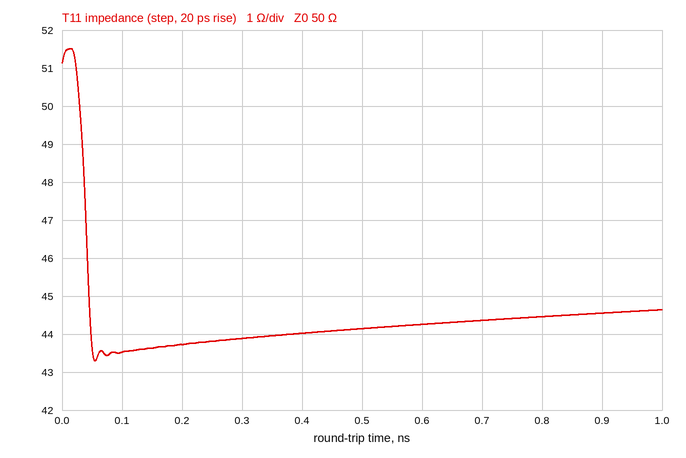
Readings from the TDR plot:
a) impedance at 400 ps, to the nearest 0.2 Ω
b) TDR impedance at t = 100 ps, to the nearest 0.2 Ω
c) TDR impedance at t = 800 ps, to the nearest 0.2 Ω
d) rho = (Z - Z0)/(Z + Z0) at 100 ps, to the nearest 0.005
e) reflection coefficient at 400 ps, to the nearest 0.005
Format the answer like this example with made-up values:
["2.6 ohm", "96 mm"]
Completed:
["44.0 Ω", "43.6 Ω", "44.4 Ω", "-0.070", "-0.065"]
